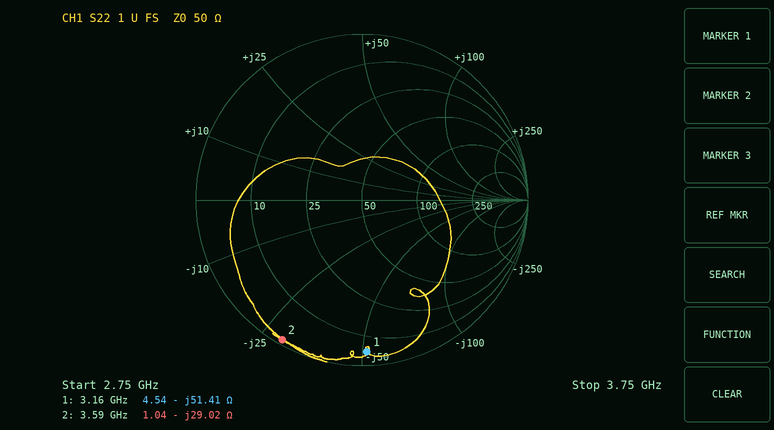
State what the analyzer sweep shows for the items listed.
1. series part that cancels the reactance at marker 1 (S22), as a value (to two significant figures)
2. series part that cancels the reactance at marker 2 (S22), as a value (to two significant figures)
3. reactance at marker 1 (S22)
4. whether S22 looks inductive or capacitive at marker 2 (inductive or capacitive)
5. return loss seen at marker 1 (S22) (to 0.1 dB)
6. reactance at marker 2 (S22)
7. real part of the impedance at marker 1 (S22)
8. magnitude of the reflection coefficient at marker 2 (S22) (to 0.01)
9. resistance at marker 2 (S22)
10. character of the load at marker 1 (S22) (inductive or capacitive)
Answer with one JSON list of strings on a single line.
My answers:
["2.6 nH", "1.3 nH", "-51.41 Ω", "capacitive", "0.8 dB", "-29.02 Ω", "4.54 Ω", "0.97", "1.04 Ω", "capacitive"]
